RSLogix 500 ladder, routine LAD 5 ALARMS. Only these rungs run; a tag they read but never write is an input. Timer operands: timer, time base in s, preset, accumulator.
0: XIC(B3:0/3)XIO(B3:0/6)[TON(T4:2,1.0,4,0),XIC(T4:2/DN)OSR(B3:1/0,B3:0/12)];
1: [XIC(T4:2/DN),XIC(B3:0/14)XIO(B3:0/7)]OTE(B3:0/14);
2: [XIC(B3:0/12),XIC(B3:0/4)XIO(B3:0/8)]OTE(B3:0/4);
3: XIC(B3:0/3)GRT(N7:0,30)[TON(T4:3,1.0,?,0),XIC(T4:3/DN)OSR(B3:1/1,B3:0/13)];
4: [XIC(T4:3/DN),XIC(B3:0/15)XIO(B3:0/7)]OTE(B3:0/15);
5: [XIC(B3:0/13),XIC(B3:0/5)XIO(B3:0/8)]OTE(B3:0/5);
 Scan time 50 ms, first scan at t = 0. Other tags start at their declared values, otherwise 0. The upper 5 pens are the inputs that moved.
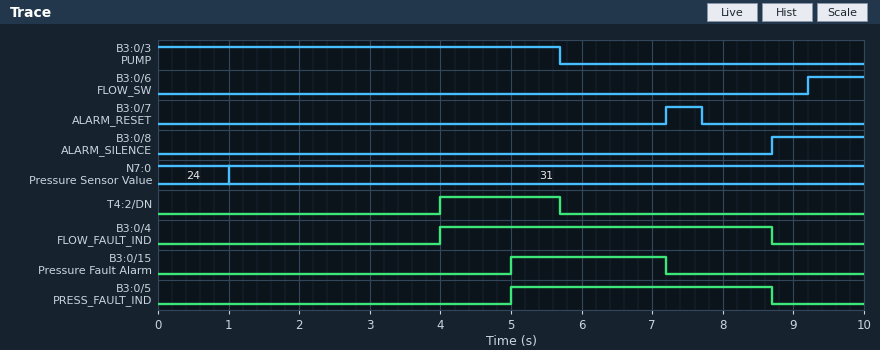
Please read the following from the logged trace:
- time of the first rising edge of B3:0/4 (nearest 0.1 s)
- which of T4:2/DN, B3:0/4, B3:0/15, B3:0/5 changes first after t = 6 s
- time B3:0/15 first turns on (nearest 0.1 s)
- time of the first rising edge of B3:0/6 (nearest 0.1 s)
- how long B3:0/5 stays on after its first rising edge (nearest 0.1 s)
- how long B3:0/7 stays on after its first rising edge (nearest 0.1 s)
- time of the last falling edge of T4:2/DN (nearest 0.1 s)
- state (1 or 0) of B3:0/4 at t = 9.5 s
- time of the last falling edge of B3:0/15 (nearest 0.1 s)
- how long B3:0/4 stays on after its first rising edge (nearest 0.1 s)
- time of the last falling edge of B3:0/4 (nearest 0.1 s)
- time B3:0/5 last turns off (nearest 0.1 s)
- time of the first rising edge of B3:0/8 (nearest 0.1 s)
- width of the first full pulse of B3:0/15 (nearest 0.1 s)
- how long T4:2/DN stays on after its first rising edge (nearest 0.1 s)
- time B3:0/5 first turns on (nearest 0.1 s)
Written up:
4.0 s
B3:0/15
5.0 s
9.2 s
3.7 s
0.5 s
5.7 s
0
7.2 s
4.7 s
8.7 s
8.7 s
8.7 s
2.2 s
1.7 s
5.0 s
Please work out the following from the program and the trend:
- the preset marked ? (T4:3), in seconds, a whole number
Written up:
4 s
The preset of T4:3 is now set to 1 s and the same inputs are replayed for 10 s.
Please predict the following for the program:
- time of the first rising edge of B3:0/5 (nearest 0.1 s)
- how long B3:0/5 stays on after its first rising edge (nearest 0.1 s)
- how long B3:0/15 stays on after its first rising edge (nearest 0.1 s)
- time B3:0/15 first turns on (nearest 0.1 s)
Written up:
2.0 s
6.7 s
5.2 s
2.0 s
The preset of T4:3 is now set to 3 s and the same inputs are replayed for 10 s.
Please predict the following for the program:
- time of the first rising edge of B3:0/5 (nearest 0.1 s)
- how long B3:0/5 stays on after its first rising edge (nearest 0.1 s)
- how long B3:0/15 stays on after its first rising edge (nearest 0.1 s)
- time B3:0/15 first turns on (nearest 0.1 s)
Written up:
4.0 s
4.7 s
3.2 s
4.0 s
